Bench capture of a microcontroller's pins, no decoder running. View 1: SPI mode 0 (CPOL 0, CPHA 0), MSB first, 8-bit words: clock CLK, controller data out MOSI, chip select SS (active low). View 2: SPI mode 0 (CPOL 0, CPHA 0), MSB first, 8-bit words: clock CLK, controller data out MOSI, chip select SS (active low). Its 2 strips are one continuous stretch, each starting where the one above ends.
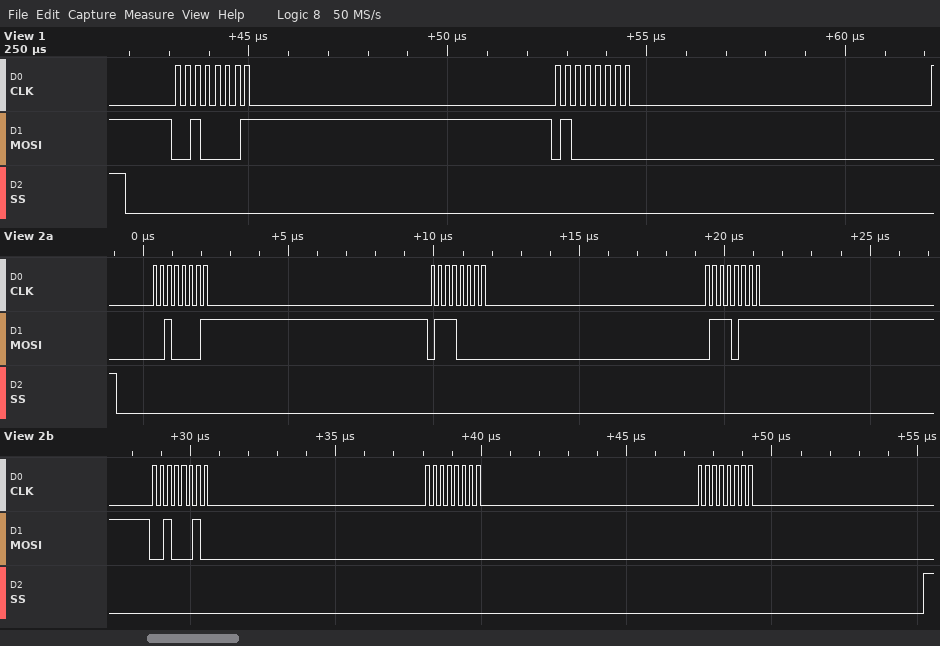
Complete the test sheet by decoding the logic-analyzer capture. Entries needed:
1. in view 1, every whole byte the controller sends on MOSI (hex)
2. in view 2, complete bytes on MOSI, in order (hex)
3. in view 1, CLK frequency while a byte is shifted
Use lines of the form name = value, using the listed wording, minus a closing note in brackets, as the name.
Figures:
in view 1, every whole byte the controller sends on MOSI = 0x21 0x40
in view 2, complete bytes on MOSI, in order = 21 70 77 22 00 00
in view 1, CLK frequency while a byte is shifted = 4 MHz
